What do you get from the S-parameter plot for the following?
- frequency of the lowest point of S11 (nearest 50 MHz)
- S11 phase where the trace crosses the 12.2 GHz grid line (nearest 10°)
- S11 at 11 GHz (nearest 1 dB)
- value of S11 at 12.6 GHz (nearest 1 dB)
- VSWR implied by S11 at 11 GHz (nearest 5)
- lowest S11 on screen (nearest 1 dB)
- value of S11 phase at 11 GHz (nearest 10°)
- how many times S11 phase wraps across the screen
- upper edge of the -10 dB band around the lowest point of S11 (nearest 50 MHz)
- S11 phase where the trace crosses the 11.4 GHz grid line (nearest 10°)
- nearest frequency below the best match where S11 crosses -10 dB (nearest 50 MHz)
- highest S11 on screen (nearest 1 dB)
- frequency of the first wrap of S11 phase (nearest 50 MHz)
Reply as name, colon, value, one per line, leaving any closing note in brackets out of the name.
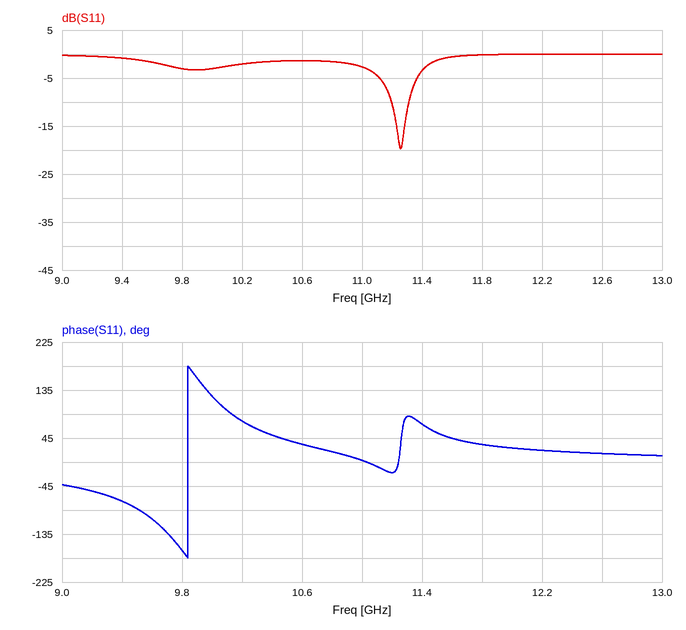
frequency of the lowest point of S11: 11.25 GHz
S11 phase where the trace crosses the 12.2 GHz grid line: 20°
S11 at 11 GHz: -3 dB
value of S11 at 12.6 GHz: 0 dB
VSWR implied by S11 at 11 GHz: 5
lowest S11 on screen: -20 dB
value of S11 phase at 11 GHz: 0°
how many times S11 phase wraps across the screen: 1
upper edge of the -10 dB band around the lowest point of S11: 11.30 GHz
S11 phase where the trace crosses the 11.4 GHz grid line: 70°
nearest frequency below the best match where S11 crosses -10 dB: 11.20 GHz
highest S11 on screen: 0 dB
frequency of the first wrap of S11 phase: 9.85 GHz
